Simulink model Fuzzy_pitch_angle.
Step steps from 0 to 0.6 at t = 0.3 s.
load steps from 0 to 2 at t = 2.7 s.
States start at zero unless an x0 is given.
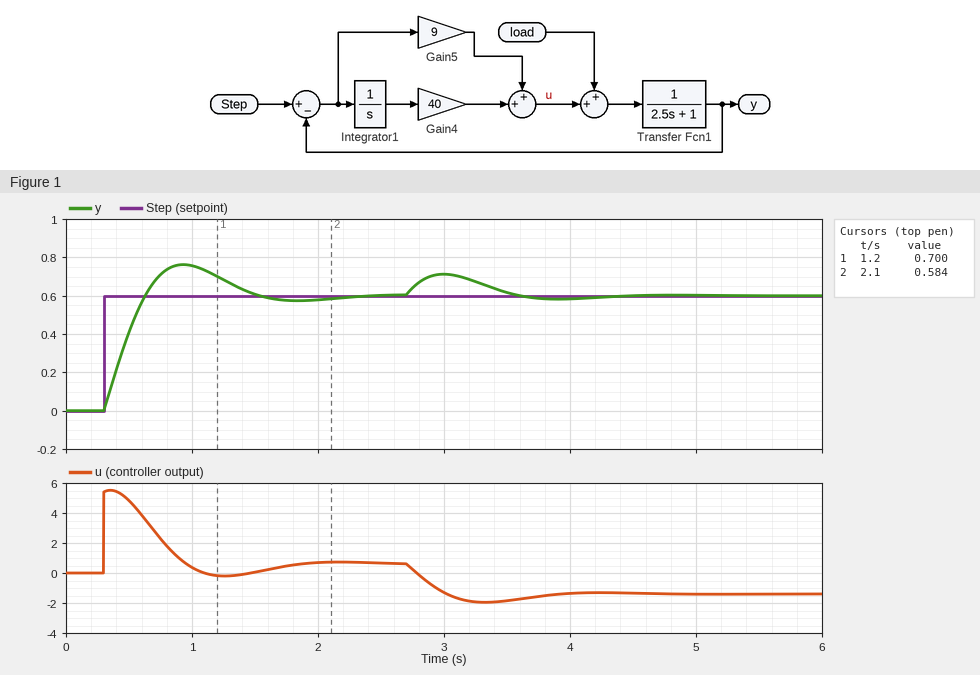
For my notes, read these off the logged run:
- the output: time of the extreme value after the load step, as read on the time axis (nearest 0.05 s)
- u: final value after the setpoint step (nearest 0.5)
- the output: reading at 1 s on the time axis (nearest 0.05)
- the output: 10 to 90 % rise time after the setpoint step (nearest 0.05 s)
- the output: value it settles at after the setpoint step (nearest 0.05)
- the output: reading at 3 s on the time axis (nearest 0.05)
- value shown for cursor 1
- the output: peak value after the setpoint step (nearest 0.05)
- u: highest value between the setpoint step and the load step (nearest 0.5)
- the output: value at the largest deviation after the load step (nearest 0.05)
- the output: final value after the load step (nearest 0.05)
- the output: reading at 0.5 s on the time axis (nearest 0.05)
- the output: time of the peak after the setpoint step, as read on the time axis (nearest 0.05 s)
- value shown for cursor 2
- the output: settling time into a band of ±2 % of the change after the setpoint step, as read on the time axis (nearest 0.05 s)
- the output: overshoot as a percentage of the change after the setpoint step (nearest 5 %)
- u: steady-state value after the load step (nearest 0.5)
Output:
3.00 s
0.5
0.75
0.25 s
0.60
0.70
0.700
0.75
5.5
0.70
0.60
0.40
0.95 s
0.584
2.20 s
25 %
-1.5
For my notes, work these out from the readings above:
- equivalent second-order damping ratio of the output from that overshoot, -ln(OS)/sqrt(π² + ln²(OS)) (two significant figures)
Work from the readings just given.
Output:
0.40
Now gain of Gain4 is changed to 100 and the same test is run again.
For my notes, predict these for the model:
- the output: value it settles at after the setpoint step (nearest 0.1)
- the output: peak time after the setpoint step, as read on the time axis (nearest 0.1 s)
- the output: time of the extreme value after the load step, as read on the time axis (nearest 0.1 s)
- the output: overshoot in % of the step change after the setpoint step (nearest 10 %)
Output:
0.6
0.7 s
2.9 s
40 %
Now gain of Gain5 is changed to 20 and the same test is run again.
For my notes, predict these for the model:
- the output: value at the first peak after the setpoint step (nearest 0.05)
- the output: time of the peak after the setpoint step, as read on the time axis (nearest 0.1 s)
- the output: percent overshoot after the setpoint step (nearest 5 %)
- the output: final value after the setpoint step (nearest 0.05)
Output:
0.65
0.8 s
10 %
0.60
